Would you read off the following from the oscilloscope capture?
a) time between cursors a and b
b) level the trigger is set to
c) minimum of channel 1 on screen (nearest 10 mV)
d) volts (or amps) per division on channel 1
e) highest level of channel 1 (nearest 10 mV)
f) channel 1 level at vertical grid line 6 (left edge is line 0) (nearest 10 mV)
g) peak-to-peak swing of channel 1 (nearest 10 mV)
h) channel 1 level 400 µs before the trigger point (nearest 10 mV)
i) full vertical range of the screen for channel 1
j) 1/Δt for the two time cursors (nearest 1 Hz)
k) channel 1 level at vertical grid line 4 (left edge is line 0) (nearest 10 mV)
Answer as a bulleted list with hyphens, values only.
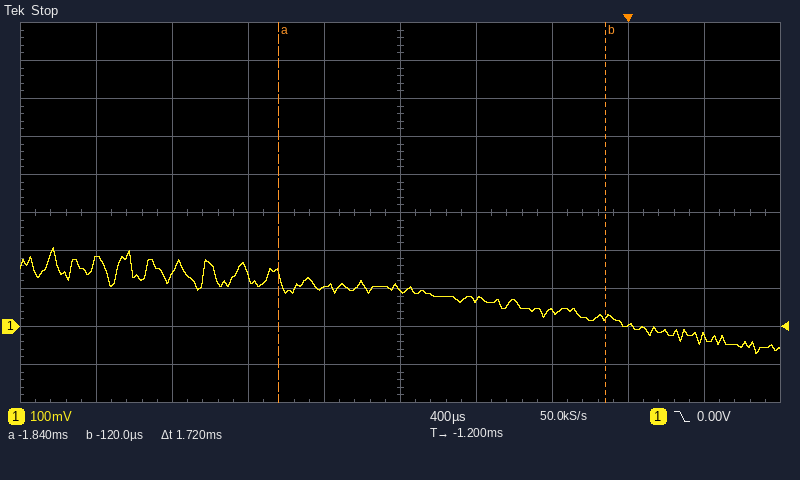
- 1.72 ms
- 0.00 V
- -70 mV
- 100 mV
- 210 mV
- 70 mV
- 280 mV
- 40 mV
- 1 V
- 581 Hz
- 100 mV
